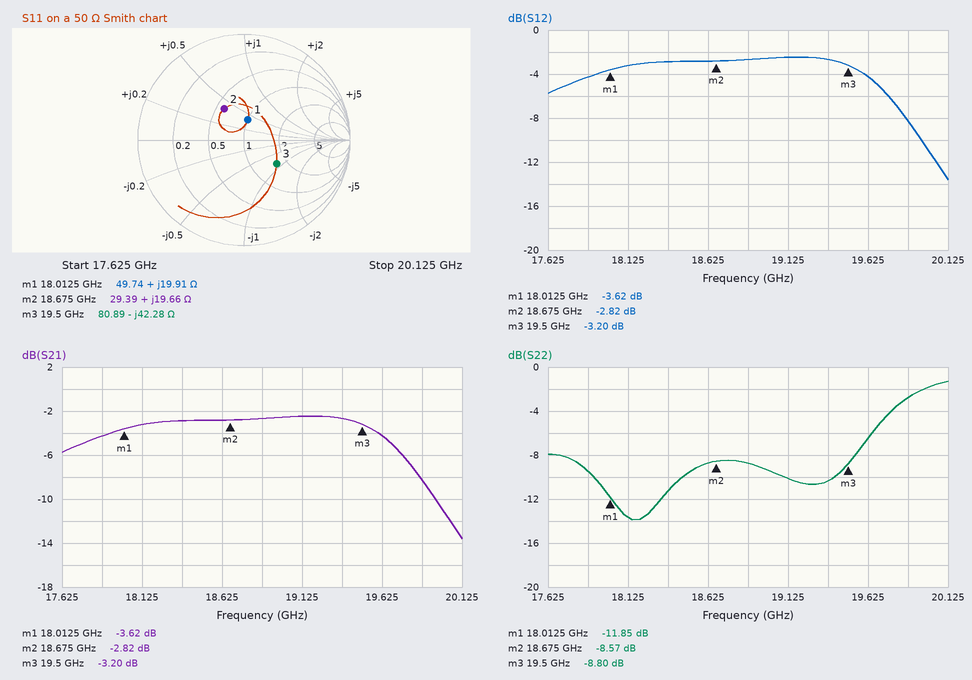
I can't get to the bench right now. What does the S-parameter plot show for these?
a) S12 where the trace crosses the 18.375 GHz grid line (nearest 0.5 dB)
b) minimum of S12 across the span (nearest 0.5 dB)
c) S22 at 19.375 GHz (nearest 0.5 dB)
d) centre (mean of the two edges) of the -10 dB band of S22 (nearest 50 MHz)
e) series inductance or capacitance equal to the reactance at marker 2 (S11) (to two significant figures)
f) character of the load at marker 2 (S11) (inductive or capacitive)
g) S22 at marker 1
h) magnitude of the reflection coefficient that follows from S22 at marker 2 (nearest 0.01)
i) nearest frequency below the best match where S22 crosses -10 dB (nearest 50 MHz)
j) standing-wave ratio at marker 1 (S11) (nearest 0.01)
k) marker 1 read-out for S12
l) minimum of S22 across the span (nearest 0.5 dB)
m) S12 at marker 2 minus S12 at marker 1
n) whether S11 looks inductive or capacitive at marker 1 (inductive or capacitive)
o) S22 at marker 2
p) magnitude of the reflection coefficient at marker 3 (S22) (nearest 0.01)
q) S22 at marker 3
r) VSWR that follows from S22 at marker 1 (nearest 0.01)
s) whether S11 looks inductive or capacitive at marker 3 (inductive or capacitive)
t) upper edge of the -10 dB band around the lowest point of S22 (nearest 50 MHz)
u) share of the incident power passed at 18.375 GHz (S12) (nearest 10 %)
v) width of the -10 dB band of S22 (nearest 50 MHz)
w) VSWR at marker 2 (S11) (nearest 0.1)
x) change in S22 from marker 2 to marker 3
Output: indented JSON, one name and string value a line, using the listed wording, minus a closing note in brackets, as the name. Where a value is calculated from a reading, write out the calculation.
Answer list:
{
  "S12 where the trace crosses the 18.375 GHz grid line": "-3.0 dB",
  "minimum of S12 across the span": "-13.5 dB",
  "S22 at 19.375 GHz": "-10.5 dB",
  "centre (mean of the two edges) of the -10 dB band of S22": "18.20 GHz",
  "series inductance or capacitance equal to the reactance at marker 2 (S11)": "L = 19.66 Ω/(2π × 18.675 GHz) ≈ 168 pH, so 170 pH to two significant figures",
  "character of the load at marker 2 (S11)": "inductive",
  "S22 at marker 1": "-11.85 dB",
  "magnitude of the reflection coefficient that follows from S22 at marker 2": "10^(-8.57/20) ≈ 0.37",
  "nearest frequency below the best match where S22 crosses -10 dB": "17.90 GHz",
  "standing-wave ratio at marker 1 (S11)": "1.49",
  "marker 1 read-out for S12": "-3.62 dB",
  "minimum of S22 across the span": "-14.0 dB",
  "S12 at marker 2 minus S12 at marker 1": "-2.82 − (-3.62) = 0.80 dB",
  "whether S11 looks inductive or capacitive at marker 1": "inductive",
  "S22 at marker 2": "-8.57 dB",
  "magnitude of the reflection coefficient at marker 3 (S22)": "10^(-8.8/20) ≈ 0.36",
  "S22 at marker 3": "-8.80 dB",
  "VSWR that follows from S22 at marker 1": "(1 + 0.2556)/(1 − 0.2556) ≈ 1.69",
  "whether S11 looks inductive or capacitive at marker 3": "capacitive",
  "upper edge of the -10 dB band around the lowest point of S22": "18.45 GHz",
  "share of the incident power passed at 18.375 GHz (S12)": "10^(-3/10) ≈ 50 %",
  "width of the -10 dB band of S22": "18.45 GHz − 17.90 GHz = 550 MHz",
  "VSWR at marker 2 (S11)": "2.1",
  "change in S22 from marker 2 to marker 3": "-8.8 − (-8.57) = -0.23 dB"
}
